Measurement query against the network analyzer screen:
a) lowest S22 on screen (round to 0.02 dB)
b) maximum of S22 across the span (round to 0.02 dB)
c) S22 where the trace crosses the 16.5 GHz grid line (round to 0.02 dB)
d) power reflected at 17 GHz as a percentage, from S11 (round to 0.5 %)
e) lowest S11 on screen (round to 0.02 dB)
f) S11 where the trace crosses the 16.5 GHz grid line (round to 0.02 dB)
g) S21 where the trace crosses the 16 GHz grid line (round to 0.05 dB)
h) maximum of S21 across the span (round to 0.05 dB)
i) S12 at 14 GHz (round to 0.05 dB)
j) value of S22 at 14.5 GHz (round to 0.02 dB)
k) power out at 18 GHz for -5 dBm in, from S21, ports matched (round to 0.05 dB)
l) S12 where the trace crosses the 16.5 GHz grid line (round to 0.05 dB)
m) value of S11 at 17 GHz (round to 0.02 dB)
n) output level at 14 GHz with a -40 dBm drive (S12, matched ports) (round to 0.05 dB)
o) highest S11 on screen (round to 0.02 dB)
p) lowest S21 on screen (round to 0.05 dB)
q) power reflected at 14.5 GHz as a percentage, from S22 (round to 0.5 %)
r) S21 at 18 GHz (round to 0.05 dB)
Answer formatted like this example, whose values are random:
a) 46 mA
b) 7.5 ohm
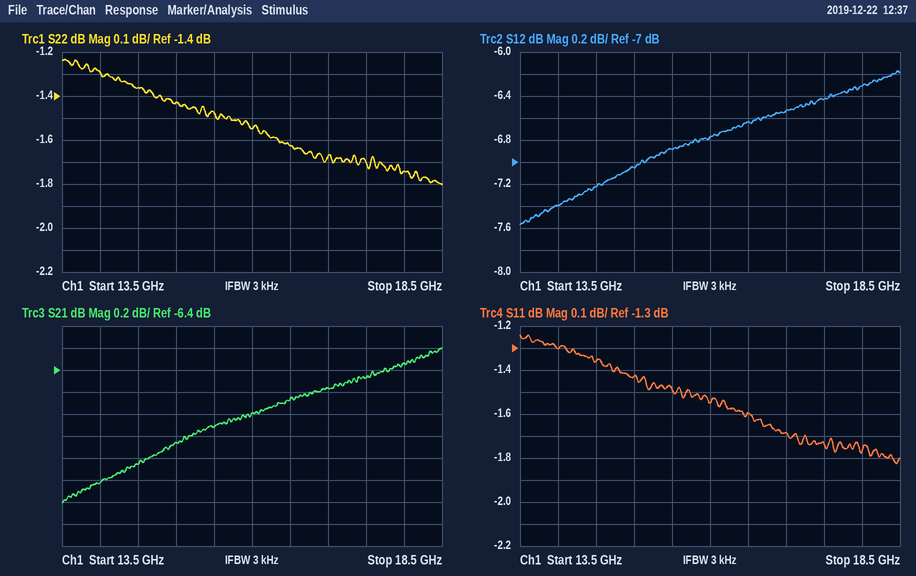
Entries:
a) -1.80 dB
b) -1.24 dB
c) -1.62 dB
d) 68.0 %
e) -1.82 dB
f) -1.60 dB
g) -6.80 dB
h) -6.20 dB
i) -7.40 dB
j) -1.36 dB
k) -11.35 dBm
l) -6.65 dB
m) -1.68 dB
n) -47.40 dBm
o) -1.24 dB
p) -7.60 dB
q) 73.0 %
r) -6.35 dB
